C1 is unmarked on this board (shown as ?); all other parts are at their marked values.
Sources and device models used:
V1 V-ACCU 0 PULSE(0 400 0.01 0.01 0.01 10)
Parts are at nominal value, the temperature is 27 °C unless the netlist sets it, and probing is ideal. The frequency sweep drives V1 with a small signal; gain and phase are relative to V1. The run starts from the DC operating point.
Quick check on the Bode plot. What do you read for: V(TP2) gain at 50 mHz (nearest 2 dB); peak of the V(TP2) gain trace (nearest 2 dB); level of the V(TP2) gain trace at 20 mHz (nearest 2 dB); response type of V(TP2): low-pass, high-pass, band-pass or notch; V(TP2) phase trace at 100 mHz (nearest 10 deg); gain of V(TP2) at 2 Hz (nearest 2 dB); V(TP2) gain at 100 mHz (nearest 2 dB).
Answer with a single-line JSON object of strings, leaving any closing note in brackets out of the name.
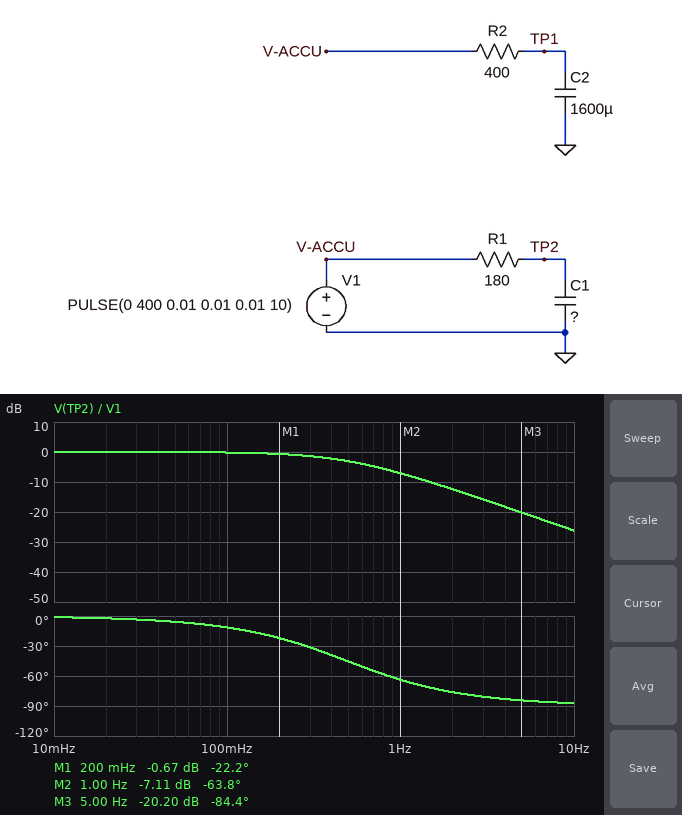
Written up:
{"V(TP2) gain at 50 mHz": "0 dB", "peak of the V(TP2) gain trace": "0 dB", "level of the V(TP2) gain trace at 20 mHz": "0 dB", "response type of V(TP2): low-pass, high-pass, band-pass or notch": "low-pass", "V(TP2) phase trace at 100 mHz": "-10 deg", "gain of V(TP2) at 2 Hz": "-12 dB", "V(TP2) gain at 100 mHz": "0 dB"}
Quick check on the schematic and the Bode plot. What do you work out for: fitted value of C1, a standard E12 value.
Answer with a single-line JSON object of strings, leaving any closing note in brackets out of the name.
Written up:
{"fitted value of C1, a standard E12 value": "1.8 mF"}
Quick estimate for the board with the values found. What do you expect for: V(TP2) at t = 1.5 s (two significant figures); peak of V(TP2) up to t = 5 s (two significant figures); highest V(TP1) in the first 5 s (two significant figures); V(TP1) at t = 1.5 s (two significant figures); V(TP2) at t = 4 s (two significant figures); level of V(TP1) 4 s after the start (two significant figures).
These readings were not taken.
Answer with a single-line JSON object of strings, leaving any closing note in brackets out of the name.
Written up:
{"V(TP2) at t = 1.5 s": "400 V", "peak of V(TP2) up to t = 5 s": "400 V", "highest V(TP1) in the first 5 s": "400 V", "V(TP1) at t = 1.5 s": "360 V", "V(TP2) at t = 4 s": "400 V", "level of V(TP1) 4 s after the start": "400 V"}
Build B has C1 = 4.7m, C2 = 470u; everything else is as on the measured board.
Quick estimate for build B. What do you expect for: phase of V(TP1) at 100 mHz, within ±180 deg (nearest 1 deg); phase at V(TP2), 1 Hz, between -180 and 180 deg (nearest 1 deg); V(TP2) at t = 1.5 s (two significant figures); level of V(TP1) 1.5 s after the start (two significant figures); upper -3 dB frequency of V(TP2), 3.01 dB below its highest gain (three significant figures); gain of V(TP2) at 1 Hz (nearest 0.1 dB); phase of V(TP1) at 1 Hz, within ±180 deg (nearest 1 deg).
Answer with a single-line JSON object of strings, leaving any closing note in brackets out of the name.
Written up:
{"phase of V(TP1) at 100 mHz, within ±180 deg": "-7 deg", "phase at V(TP2), 1 Hz, between -180 and 180 deg": "-79 deg", "V(TP2) at t = 1.5 s": "330 V", "level of V(TP1) 1.5 s after the start": "400 V", "upper -3 dB frequency of V(TP2), 3.01 dB below its highest gain": "188 mHz", "gain of V(TP2) at 1 Hz": "-14.7 dB", "phase of V(TP1) at 1 Hz, within ±180 deg": "-50 deg"}
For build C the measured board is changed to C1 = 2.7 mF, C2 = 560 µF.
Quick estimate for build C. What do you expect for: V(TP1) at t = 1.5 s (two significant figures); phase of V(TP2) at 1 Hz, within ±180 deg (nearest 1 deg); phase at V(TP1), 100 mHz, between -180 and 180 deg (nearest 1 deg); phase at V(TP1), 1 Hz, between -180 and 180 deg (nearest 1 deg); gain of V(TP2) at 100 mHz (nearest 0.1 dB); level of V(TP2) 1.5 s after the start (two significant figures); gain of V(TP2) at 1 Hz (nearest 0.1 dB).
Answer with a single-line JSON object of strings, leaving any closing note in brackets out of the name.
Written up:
{"V(TP1) at t = 1.5 s": "400 V", "phase of V(TP2) at 1 Hz, within ±180 deg": "-72 deg", "phase at V(TP1), 100 mHz, between -180 and 180 deg": "-8 deg", "phase at V(TP1), 1 Hz, between -180 and 180 deg": "-55 deg", "gain of V(TP2) at 100 mHz": "-0.4 dB", "level of V(TP2) 1.5 s after the start": "380 V", "gain of V(TP2) at 1 Hz": "-10.1 dB"}
